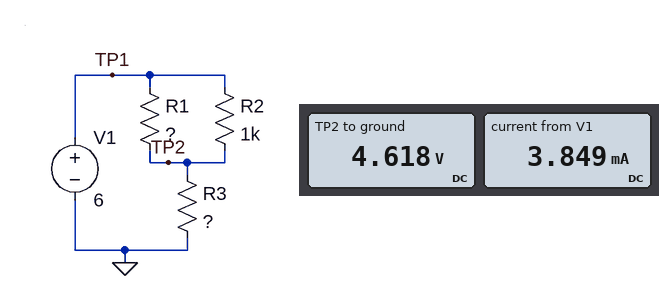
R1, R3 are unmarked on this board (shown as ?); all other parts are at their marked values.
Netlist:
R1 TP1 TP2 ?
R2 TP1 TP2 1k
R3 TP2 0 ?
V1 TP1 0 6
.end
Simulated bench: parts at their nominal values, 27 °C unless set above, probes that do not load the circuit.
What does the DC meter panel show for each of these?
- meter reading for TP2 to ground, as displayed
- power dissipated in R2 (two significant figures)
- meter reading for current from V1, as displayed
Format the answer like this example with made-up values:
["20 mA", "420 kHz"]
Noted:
["4.618 V", "1.9 mW", "3.849 mA"]
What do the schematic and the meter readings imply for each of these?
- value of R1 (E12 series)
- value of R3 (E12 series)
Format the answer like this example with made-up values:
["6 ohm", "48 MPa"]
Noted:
["560 Ω", "1.2 kΩ"]
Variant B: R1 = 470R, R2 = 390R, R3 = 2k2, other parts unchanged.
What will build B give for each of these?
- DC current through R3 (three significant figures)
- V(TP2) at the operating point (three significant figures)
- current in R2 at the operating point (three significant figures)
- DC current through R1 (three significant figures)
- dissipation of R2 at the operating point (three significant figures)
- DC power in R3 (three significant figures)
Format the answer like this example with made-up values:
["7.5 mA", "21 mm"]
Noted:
["2.49 mA", "5.47 V", "1.36 mA", "1.13 mA", "720 µW", "13.6 mW"]
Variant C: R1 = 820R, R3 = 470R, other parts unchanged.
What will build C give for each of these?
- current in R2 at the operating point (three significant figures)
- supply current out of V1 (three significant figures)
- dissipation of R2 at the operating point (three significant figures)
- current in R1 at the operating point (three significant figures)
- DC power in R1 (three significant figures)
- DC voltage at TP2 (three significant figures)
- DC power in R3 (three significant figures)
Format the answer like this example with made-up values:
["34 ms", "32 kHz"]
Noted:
["2.94 mA", "6.52 mA", "8.62 mW", "3.58 mA", "10.5 mW", "3.06 V", "20.0 mW"]
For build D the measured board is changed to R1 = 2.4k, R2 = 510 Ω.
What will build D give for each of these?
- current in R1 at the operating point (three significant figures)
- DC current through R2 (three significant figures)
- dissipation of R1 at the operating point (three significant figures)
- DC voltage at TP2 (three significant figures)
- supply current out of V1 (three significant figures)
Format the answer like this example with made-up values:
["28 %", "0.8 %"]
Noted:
["649 µA", "3.05 mA", "1.01 mW", "4.44 V", "3.70 mA"]
